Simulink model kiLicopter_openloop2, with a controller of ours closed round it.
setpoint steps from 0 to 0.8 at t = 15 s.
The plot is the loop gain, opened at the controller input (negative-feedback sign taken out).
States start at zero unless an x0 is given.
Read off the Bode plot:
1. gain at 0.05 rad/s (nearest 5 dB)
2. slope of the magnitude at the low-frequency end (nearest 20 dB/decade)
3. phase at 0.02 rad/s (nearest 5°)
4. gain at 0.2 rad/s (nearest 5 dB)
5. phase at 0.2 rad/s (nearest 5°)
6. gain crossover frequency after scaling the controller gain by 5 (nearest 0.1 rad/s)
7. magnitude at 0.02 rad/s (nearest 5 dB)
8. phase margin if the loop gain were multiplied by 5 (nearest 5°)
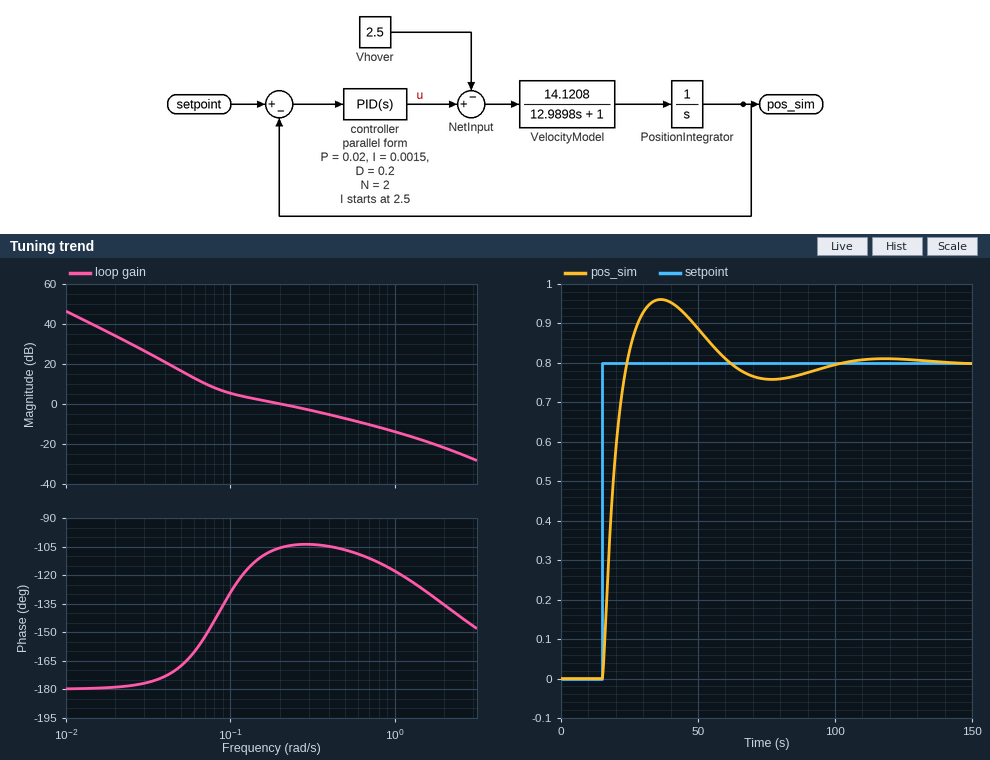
15 dB
-40 dB/decade
-180°
0 dB
-105°
1.0 rad/s
35 dB
60°
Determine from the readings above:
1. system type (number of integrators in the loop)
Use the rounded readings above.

2
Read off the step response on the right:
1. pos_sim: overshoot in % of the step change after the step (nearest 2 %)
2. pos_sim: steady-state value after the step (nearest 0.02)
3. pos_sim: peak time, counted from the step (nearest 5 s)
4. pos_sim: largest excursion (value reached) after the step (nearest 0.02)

20 %
0.80
20 s
0.96
